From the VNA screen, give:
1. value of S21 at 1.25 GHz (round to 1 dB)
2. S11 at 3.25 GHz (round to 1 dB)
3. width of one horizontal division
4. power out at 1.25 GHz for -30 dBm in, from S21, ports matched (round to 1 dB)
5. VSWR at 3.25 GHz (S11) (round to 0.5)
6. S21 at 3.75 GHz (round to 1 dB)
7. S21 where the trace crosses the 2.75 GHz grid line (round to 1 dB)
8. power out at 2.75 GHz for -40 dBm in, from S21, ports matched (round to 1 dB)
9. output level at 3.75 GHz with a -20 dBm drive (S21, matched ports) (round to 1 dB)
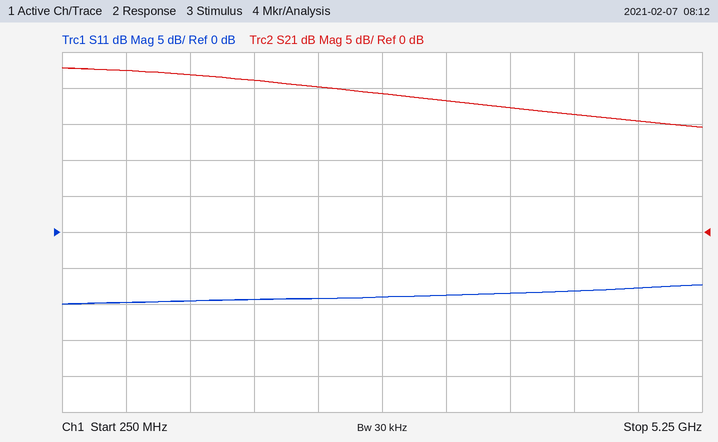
22 dB
-9 dB
500 MHz
-8 dBm
2.0
17 dB
19 dB
-21 dBm
-3 dBm
